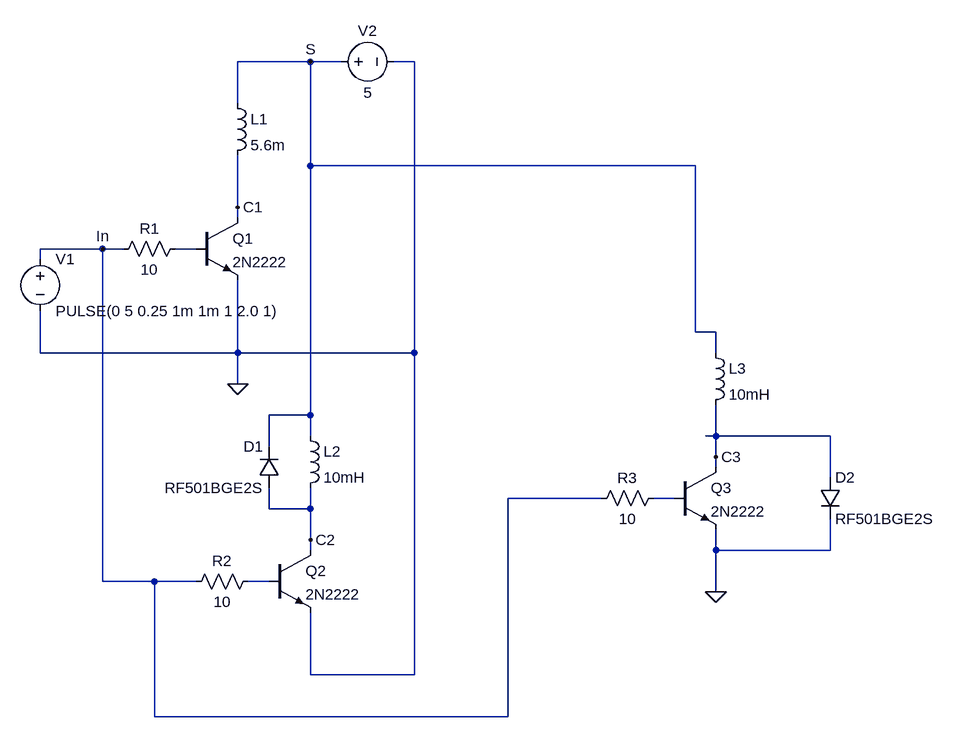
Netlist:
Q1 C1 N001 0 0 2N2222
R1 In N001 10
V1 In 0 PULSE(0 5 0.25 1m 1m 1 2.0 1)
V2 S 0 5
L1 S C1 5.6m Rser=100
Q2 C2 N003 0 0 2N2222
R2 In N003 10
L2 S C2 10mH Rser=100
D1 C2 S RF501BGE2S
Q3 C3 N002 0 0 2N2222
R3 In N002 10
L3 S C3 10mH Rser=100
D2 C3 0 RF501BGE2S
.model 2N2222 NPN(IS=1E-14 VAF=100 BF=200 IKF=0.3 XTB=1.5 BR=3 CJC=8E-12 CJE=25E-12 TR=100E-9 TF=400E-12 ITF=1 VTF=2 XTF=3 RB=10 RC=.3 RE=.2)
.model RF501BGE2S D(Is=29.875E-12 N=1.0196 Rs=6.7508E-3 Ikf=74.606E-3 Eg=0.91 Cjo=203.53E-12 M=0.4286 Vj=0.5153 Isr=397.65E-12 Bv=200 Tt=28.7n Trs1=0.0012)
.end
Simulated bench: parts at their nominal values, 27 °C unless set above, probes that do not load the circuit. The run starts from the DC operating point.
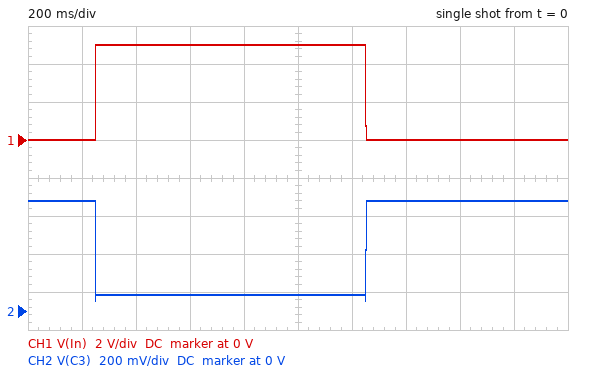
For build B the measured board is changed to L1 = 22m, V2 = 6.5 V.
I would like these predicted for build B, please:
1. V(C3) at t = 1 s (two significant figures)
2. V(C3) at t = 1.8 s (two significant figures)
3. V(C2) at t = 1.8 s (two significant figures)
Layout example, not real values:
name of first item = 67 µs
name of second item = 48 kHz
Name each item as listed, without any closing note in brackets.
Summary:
V(C3) at t = 1 s = 93 mV
V(C3) at t = 1.8 s = 590 mV
V(C2) at t = 1.8 s = 6.5 V
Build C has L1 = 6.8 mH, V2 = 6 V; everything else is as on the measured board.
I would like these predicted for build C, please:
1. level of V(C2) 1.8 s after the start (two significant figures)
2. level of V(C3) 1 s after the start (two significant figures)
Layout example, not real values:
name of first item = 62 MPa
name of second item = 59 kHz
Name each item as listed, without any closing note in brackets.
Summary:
level of V(C2) 1.8 s after the start = 6.0 V
level of V(C3) 1 s after the start = 90 mV
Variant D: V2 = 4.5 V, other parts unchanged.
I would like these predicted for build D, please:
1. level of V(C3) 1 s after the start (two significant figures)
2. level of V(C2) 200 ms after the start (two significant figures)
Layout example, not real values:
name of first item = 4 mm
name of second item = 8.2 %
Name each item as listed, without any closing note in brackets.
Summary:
level of V(C3) 1 s after the start = 82 mV
level of V(C2) 200 ms after the start = 4.5 V
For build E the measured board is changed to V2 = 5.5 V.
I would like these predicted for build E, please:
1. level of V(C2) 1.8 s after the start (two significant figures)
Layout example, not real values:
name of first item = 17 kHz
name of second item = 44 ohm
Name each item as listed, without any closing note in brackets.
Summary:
level of V(C2) 1.8 s after the start = 5.5 V
